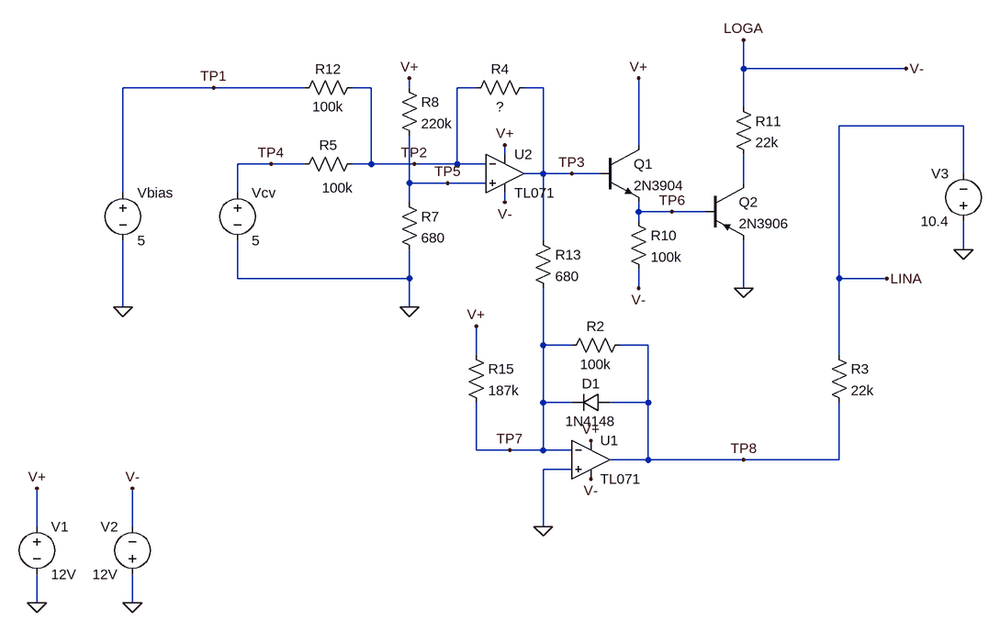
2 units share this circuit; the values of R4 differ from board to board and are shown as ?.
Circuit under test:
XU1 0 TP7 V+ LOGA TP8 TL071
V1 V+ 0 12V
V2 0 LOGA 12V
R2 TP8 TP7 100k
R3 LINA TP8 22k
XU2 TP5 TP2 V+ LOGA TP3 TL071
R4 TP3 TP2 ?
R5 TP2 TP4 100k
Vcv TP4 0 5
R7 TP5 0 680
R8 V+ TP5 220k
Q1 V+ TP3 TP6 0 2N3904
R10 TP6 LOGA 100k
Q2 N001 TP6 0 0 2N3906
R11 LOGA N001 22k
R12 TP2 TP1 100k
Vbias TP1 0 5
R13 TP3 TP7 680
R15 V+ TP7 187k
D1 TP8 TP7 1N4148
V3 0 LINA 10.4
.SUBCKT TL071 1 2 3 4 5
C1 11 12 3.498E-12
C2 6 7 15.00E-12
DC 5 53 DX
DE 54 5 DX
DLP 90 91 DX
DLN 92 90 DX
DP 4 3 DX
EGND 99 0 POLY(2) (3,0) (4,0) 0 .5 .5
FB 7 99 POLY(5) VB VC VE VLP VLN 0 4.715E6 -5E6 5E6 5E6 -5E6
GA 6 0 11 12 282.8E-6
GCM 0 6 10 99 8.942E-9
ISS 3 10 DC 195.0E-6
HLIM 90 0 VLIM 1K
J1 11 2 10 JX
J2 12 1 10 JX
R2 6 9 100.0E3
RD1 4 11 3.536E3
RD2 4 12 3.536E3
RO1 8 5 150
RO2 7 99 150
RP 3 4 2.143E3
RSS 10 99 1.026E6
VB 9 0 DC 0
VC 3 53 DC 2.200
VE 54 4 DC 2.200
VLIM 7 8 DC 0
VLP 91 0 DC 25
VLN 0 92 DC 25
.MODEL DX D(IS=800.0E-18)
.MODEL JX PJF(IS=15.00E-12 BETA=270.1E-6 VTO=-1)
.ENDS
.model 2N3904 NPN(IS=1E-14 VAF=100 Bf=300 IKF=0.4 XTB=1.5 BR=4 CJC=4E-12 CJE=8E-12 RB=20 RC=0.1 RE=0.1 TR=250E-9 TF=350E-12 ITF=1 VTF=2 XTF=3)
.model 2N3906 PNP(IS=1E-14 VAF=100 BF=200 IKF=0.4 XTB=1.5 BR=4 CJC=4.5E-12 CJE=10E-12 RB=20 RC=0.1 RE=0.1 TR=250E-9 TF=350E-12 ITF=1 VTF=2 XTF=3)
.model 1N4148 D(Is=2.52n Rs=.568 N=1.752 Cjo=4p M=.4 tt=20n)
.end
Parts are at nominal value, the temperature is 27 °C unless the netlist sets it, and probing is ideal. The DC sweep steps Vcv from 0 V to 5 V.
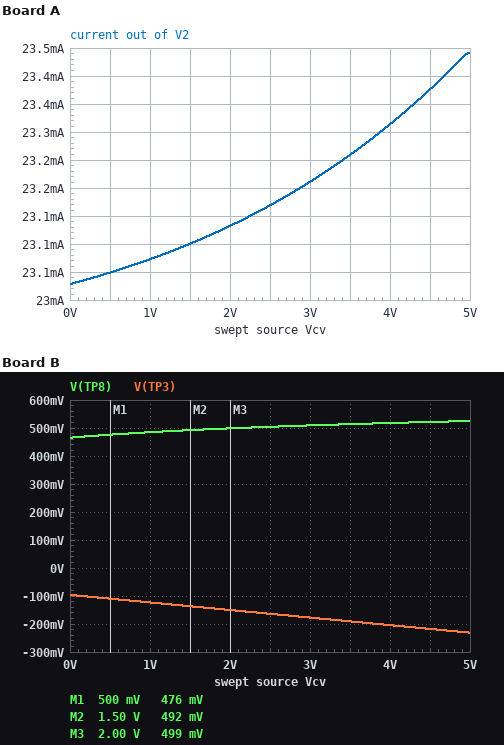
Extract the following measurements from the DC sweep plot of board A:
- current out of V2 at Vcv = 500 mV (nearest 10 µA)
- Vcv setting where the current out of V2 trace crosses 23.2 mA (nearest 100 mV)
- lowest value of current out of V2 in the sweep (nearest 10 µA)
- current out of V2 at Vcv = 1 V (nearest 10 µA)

23.05 mA
3.4 V
23.03 mA
23.07 mA
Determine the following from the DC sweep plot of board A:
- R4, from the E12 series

820 Ω
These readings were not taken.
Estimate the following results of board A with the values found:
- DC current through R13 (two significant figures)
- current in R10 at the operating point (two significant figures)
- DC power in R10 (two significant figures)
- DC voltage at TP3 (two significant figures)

65 µA
110 µA
1.3 mW
-44 mV
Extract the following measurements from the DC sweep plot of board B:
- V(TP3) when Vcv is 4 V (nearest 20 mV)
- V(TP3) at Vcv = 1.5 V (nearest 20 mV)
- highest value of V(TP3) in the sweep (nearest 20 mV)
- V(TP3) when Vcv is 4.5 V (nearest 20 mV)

-200 mV
-140 mV
-100 mV
-220 mV
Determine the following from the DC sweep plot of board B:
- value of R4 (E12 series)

2.7 kΩ
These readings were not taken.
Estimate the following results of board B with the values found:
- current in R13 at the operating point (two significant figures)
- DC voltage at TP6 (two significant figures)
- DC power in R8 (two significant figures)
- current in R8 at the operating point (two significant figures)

340 µA
-660 mV
650 µW
54 µA
